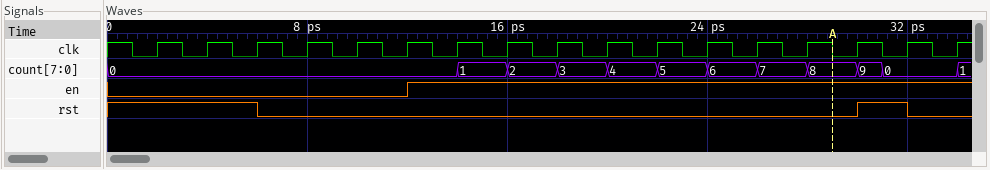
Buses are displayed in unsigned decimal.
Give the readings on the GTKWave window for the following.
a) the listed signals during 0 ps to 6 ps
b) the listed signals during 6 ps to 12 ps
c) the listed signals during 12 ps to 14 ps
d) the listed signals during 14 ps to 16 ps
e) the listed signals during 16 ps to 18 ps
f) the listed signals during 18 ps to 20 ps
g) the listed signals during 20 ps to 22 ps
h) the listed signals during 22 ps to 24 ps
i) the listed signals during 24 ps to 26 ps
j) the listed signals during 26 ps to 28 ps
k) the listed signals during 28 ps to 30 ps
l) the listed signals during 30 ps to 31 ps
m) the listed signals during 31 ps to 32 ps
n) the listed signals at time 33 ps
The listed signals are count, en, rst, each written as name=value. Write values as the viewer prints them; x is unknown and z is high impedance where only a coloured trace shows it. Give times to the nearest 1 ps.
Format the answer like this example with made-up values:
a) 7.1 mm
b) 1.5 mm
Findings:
a) count=0, en=0, rst=1
b) count=0, en=0, rst=0
c) count=0, en=1, rst=0
d) count=1, en=1, rst=0
e) count=2, en=1, rst=0
f) count=3, en=1, rst=0
g) count=4, en=1, rst=0
h) count=5, en=1, rst=0
i) count=6, en=1, rst=0
j) count=7, en=1, rst=0
k) count=8, en=1, rst=0
l) count=9, en=1, rst=1
m) count=0, en=1, rst=1
n) count=0, en=1, rst=0
